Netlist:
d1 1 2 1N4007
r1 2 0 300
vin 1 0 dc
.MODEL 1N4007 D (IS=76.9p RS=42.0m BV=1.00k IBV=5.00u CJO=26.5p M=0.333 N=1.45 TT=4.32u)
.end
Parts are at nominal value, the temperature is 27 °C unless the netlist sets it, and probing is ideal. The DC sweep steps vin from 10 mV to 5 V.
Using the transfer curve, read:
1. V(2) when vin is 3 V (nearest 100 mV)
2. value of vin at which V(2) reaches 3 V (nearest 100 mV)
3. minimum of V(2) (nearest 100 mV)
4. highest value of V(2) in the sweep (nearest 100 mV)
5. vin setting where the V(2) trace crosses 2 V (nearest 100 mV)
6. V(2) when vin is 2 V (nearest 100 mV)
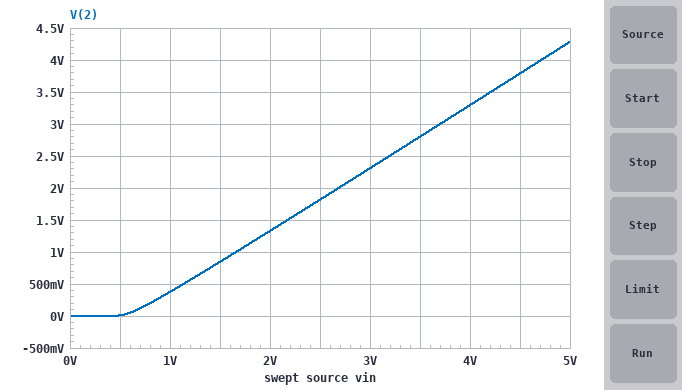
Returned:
2.3 V
3.7 V
0 V
4.3 V
2.7 V
1.3 V
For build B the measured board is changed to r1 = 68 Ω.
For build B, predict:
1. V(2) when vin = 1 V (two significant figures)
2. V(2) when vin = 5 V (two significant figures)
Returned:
330 mV
4.2 V
